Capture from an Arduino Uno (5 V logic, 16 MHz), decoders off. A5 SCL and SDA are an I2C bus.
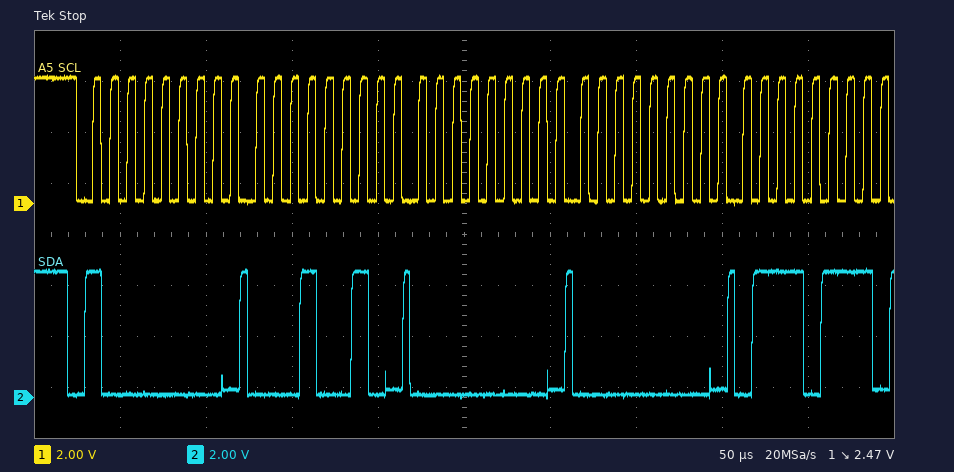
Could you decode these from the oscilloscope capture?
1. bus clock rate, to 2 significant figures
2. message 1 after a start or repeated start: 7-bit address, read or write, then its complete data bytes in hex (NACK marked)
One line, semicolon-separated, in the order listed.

100 kHz; 0x40 write: 12 00 00 77
